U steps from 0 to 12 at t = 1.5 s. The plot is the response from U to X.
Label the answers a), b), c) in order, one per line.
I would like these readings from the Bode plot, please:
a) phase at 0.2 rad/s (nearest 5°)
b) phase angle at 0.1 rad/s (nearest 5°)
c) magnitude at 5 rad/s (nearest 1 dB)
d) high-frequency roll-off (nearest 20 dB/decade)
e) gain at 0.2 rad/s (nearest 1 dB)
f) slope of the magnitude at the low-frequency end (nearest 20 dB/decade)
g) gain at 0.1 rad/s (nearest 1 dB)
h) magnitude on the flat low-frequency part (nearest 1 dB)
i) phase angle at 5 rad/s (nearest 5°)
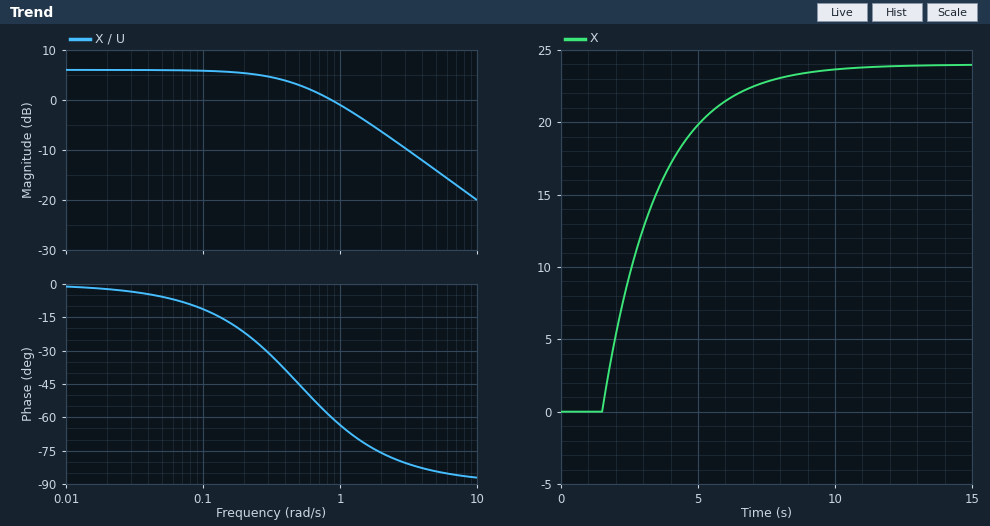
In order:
a) -20°
b) -10°
c) -14 dB
d) -20 dB/decade
e) 5 dB
f) 0 dB/decade
g) 6 dB
h) 6 dB
i) -85°
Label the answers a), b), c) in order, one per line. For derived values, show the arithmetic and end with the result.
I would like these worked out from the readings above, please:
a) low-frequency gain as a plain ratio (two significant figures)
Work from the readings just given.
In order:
a) 10^(6 / 20) = 2.0
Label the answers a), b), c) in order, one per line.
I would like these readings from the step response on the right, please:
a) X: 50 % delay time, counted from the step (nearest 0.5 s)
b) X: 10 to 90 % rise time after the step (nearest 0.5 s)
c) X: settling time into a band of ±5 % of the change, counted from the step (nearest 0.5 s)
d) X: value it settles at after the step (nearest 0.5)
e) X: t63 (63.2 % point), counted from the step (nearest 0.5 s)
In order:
a) 1.5 s
b) 4.5 s
c) 6.0 s
d) 24.0
e) 2.0 s
